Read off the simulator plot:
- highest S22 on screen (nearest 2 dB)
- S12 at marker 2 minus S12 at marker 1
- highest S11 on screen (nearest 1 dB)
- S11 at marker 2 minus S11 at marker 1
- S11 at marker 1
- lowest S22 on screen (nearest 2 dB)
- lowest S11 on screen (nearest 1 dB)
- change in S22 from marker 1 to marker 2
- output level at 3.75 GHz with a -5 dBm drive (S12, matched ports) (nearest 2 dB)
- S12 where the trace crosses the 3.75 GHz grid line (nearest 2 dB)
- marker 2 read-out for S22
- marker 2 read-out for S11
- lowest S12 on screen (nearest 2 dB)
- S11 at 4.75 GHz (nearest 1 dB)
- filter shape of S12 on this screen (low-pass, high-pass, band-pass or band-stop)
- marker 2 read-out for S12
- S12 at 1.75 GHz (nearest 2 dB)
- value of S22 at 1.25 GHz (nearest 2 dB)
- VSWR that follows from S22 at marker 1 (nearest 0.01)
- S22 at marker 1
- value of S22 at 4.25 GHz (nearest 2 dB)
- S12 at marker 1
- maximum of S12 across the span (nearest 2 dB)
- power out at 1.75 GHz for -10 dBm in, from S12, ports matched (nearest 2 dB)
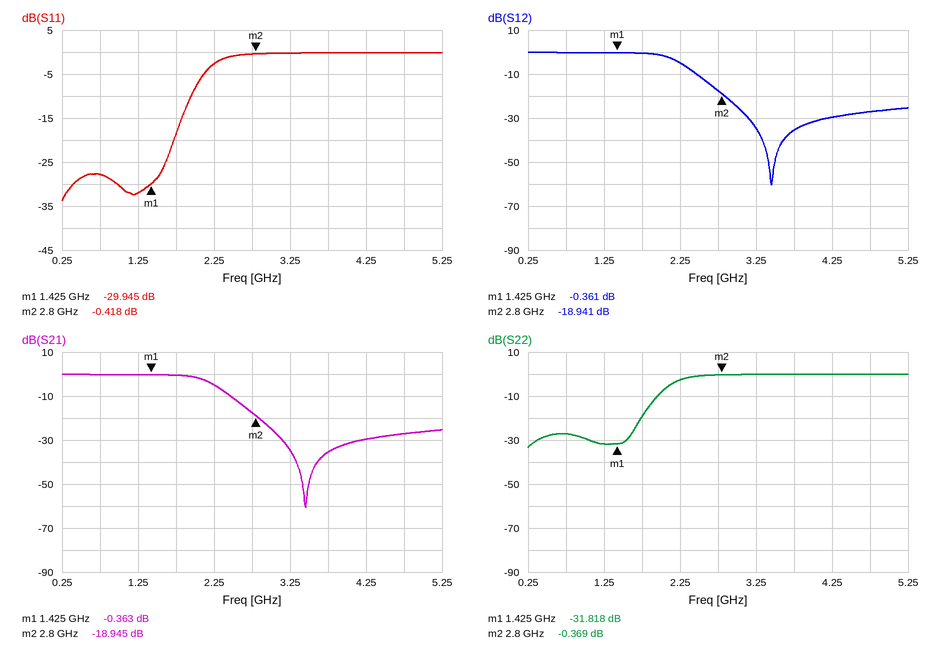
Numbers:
0 dB
-18.580 dB
0 dB
29.527 dB
-29.945 dB
-34 dB
-34 dB
31.449 dB
-40 dBm
-36 dB
-0.369 dB
-0.418 dB
-60 dB
0 dB
low-pass
-18.941 dB
0 dB
-32 dB
1.05
-31.818 dB
0 dB
-0.361 dB
0 dB
-10 dBm
